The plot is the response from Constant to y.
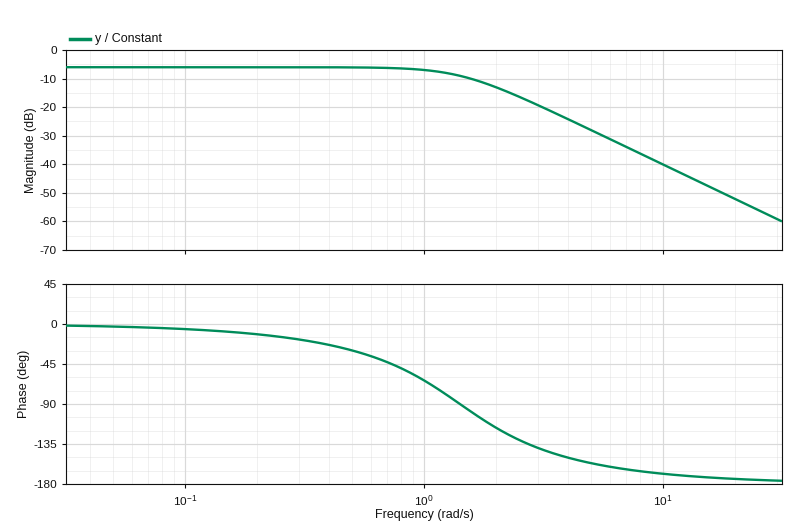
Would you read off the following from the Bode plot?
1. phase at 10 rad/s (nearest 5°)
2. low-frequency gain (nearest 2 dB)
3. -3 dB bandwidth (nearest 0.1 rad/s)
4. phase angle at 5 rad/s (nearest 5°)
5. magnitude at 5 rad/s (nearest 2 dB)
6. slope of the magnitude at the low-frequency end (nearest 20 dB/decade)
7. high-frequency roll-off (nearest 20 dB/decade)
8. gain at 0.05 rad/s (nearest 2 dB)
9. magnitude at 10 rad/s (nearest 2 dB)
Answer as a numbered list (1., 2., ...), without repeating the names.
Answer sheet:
1. -170°
2. -6 dB
3. 1.4 rad/s
4. -155°
5. -28 dB
6. 0 dB/decade
7. -40 dB/decade
8. -6 dB
9. -40 dB
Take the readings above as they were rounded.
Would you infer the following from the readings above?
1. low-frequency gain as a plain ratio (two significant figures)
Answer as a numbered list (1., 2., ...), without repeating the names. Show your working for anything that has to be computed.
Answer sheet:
1. 10^(-6 / 20) = 0.50
